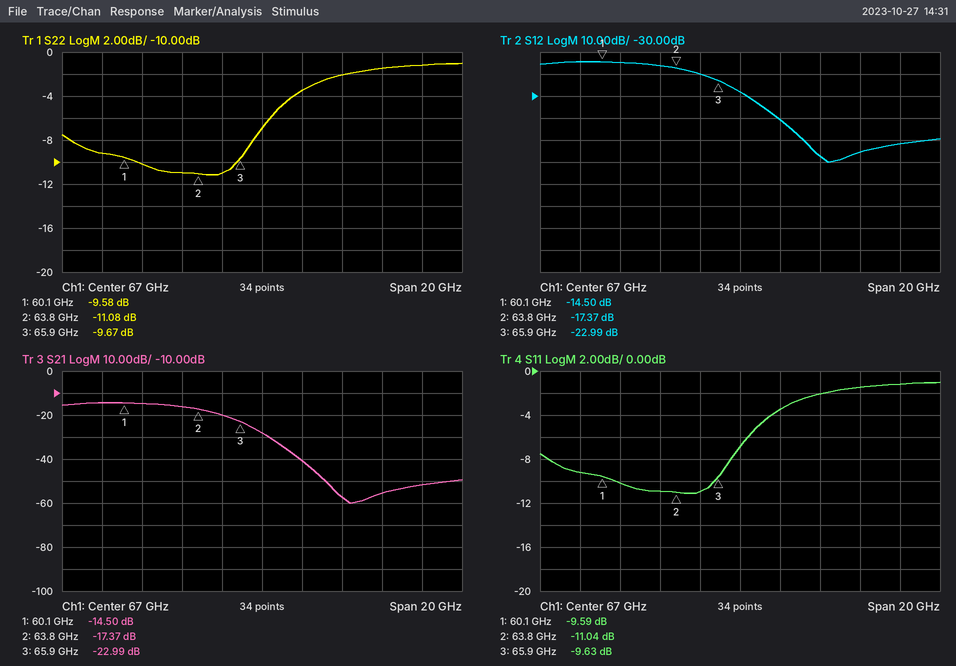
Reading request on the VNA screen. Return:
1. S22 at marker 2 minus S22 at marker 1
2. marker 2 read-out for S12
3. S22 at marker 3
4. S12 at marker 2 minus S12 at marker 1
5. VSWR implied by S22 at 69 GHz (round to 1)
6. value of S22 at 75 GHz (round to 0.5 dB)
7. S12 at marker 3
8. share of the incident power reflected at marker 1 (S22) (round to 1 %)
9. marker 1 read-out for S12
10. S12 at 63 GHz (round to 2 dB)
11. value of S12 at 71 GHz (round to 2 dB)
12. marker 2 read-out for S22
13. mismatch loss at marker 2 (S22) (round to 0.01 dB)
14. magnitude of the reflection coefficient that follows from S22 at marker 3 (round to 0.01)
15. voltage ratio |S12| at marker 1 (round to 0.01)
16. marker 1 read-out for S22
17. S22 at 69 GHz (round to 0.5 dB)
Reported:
-1.50 dB
-17.37 dB
-9.67 dB
-2.87 dB
5
-1.0 dB
-22.99 dB
11 %
-14.50 dB
-16 dB
-58 dB
-11.08 dB
0.35 dB
0.33
0.19
-9.58 dB
-3.5 dB
